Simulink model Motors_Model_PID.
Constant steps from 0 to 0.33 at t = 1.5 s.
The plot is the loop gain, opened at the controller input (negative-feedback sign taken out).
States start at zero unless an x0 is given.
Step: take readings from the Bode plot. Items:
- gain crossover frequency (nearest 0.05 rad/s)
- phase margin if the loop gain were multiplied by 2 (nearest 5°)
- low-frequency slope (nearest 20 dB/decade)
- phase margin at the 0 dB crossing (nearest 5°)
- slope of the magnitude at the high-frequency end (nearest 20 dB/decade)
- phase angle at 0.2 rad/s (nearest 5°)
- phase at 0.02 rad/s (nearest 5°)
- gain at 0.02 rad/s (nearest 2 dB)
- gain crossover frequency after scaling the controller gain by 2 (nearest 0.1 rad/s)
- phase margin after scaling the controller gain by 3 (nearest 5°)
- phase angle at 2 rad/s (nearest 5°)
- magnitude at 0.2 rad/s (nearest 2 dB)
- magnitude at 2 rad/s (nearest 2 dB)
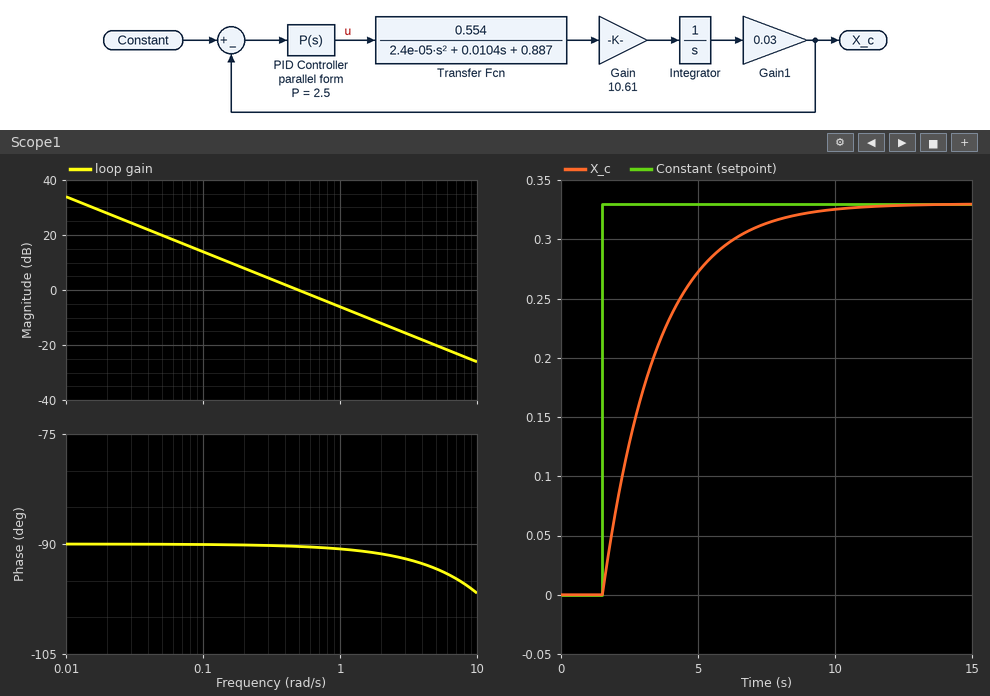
0.50 rad/s
90°
-20 dB/decade
90°
-20 dB/decade
-90°
-90°
28 dB
1.0 rad/s
90°
-90°
8 dB
-12 dB
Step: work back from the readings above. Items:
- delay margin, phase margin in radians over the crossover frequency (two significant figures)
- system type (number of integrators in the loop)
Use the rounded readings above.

3.1 s
1
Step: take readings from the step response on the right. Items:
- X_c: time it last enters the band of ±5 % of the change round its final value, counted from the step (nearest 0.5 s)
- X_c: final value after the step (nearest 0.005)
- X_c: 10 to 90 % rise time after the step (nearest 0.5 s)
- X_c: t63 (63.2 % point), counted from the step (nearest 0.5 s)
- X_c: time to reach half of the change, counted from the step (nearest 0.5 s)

6.0 s
0.330
4.5 s
2.0 s
1.5 s
